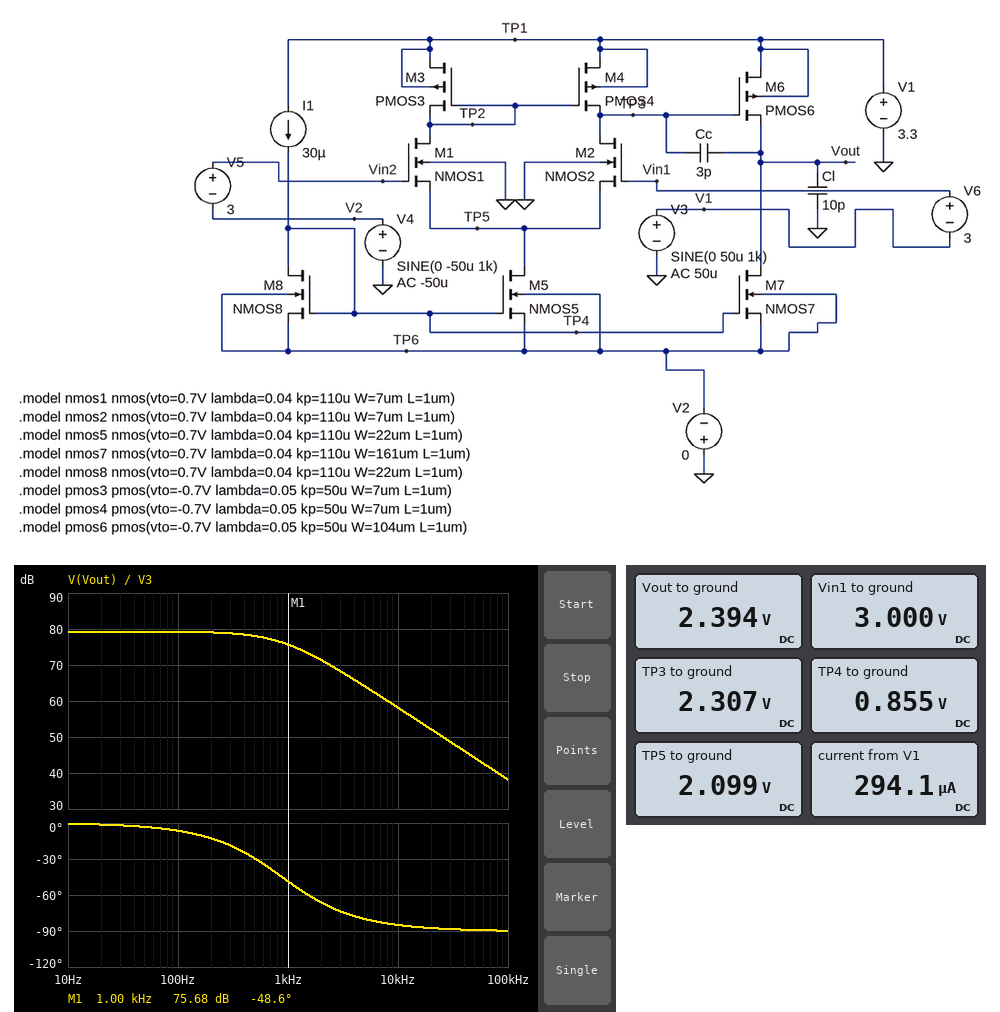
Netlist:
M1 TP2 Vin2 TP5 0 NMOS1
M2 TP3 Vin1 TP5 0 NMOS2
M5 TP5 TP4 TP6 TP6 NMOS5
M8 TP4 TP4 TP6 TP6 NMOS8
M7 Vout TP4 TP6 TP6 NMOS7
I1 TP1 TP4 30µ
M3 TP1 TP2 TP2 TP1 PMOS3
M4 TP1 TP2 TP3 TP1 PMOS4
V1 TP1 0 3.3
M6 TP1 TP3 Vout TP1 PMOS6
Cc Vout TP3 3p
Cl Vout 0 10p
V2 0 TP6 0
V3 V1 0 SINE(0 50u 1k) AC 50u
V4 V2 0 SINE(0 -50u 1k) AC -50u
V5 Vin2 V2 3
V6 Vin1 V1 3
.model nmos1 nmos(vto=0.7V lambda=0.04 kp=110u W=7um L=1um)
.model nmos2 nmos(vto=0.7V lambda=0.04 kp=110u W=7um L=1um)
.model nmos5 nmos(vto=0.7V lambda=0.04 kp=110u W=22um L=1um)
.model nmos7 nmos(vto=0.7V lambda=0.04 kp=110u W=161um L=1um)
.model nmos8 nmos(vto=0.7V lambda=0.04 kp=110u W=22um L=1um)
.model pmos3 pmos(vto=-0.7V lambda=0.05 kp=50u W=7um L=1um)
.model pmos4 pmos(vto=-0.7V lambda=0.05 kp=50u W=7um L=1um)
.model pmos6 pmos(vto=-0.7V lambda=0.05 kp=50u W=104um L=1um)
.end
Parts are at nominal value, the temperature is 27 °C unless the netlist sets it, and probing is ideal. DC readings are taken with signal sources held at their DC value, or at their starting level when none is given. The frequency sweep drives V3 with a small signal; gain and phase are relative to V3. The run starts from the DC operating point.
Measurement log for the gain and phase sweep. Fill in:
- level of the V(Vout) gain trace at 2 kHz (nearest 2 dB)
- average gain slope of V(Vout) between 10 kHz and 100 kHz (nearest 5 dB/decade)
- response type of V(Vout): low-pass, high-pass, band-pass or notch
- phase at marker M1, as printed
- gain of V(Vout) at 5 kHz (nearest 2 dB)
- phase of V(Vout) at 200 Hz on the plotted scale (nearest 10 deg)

72 dB
-20 dB/decade
low-pass
-48.6 deg
64 dB
-10 deg
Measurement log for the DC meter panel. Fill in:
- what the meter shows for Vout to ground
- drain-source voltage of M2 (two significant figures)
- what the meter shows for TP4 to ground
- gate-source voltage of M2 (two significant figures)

2.394 V
210 mV
0.855 V
900 mV
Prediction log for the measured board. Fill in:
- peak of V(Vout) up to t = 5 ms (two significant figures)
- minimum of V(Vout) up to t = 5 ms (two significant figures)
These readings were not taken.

3.0 V
1.8 V
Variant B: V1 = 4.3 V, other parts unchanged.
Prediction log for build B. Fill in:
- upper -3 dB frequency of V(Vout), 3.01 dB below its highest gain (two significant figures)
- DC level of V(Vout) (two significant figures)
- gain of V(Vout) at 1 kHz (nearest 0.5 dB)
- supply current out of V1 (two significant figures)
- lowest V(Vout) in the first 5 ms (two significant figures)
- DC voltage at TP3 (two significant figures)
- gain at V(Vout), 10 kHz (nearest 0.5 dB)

850 Hz
3.0 V
76.0 dB
300 µA
2.3 V
3.3 V
58.5 dB
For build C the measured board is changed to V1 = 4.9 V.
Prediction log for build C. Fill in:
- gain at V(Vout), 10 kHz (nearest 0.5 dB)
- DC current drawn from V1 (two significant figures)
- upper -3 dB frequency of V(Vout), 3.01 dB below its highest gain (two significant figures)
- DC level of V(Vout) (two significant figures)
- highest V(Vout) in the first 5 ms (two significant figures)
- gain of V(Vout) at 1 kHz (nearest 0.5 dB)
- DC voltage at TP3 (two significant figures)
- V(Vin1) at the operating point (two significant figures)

58.5 dB
300 µA
830 Hz
3.3 V
4.0 V
76.0 dB
3.9 V
3.0 V
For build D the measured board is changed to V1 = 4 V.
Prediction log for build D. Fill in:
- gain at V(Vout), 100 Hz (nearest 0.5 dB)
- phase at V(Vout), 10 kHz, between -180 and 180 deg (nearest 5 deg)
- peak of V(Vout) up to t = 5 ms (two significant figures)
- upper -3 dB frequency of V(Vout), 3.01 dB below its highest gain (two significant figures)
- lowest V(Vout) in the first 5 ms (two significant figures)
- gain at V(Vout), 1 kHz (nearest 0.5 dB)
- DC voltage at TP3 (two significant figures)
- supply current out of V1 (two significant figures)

79.5 dB
-85 deg
3.5 V
860 Hz
2.2 V
76.0 dB
3.0 V
300 µA
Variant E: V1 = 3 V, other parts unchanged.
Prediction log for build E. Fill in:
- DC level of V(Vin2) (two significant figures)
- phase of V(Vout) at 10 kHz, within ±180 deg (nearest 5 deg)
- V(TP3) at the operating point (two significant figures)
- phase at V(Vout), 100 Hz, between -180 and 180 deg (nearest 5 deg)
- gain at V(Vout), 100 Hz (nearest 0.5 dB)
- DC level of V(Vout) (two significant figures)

3.0 V
-10 deg
2.0 V
0 deg
24.5 dB
2.2 V
